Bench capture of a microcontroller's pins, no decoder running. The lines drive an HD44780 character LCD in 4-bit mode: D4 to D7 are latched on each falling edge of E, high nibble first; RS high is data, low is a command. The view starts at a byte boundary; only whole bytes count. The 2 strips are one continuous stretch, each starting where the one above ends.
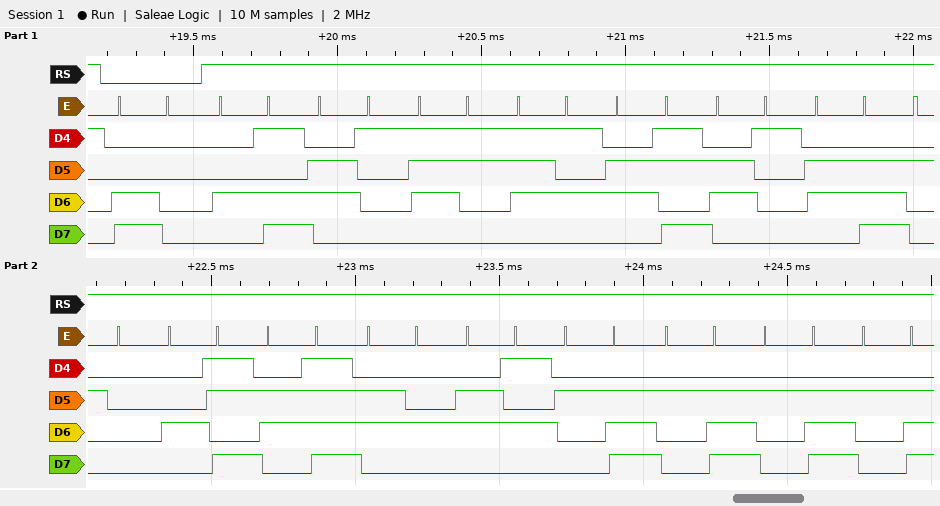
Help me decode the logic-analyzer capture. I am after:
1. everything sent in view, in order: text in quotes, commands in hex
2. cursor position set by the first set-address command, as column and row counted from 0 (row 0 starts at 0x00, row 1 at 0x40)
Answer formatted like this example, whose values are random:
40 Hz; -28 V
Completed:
0xC0 "Masukan Kode...."; column 0, row 1
